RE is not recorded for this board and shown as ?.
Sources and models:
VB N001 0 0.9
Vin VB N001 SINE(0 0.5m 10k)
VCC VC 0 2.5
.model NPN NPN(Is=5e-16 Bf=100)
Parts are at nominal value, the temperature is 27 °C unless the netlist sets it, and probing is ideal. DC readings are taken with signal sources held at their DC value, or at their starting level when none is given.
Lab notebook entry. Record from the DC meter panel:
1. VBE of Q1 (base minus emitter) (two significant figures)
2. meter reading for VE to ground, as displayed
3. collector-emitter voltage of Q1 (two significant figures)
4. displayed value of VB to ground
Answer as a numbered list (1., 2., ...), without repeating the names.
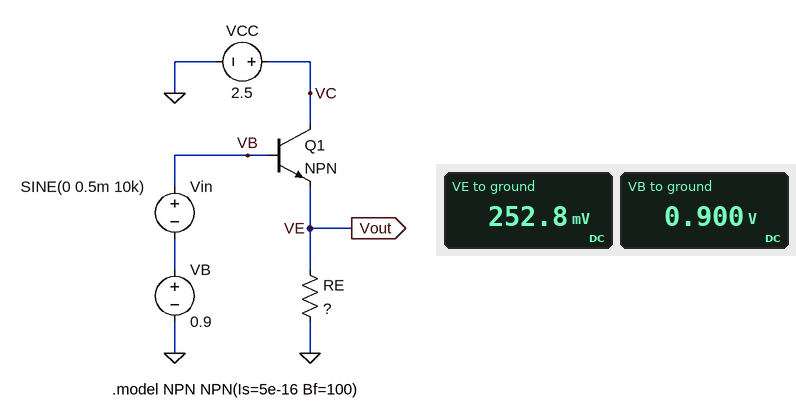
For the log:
1. 650 mV
2. 252.8 mV
3. 2.2 V
4. 0.900 V
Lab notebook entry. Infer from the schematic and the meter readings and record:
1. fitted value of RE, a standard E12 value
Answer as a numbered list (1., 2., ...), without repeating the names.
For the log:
1. 6.8 kΩ
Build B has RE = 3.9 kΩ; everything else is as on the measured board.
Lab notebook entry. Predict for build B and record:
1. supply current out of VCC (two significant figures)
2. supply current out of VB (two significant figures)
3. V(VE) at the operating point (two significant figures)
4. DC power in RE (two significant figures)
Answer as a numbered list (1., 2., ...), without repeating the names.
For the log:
1. 61 µA
2. 610 nA
3. 240 mV
4. 15 µW
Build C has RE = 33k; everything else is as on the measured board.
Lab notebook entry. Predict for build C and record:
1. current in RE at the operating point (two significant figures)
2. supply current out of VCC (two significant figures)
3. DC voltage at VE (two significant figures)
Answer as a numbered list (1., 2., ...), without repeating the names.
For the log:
1. 8.8 µA
2. 8.7 µA
3. 290 mV
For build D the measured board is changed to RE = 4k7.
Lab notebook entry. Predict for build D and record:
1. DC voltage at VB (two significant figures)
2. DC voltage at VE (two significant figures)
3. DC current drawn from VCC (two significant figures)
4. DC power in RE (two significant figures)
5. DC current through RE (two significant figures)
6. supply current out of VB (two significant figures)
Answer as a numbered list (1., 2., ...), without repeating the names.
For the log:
1. 900 mV
2. 240 mV
3. 51 µA
4. 13 µW
5. 52 µA
6. 510 nA
